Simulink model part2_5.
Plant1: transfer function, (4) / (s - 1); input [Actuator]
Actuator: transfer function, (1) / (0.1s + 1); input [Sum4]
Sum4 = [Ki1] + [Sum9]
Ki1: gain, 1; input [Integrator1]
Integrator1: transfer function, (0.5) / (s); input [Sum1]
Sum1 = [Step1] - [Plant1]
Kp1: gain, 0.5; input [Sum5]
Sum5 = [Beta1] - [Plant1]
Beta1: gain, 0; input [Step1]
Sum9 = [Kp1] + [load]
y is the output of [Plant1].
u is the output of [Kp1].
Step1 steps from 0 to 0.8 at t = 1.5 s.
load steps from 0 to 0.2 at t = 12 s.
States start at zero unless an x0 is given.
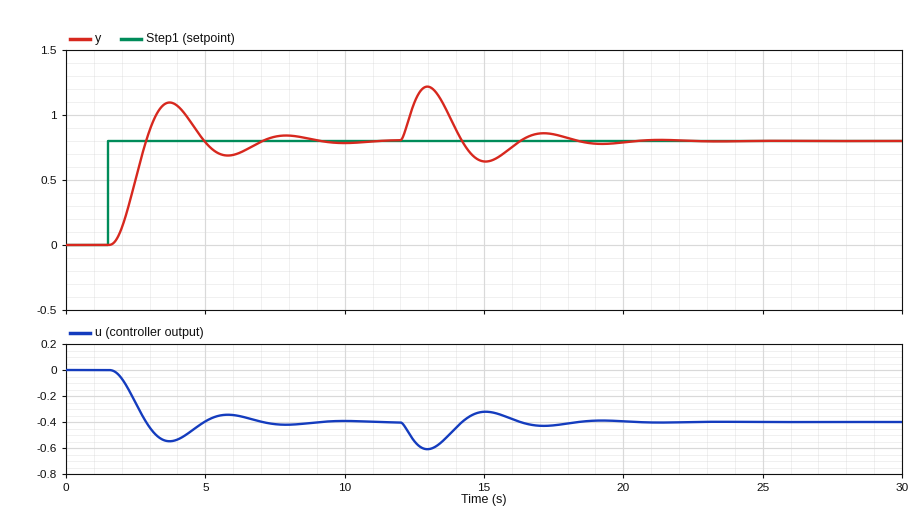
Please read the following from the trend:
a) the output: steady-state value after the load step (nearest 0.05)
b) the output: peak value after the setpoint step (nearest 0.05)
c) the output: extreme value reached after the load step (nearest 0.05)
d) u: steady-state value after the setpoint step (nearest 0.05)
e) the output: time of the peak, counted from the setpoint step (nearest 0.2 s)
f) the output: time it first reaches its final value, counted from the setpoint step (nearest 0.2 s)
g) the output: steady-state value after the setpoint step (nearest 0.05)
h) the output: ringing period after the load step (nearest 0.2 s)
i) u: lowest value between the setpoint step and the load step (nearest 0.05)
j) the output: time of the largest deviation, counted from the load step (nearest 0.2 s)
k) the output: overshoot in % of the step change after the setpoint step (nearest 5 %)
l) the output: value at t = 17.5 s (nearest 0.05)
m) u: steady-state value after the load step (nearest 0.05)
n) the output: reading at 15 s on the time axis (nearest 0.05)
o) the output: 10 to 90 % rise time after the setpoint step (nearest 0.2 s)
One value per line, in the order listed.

0.80
1.10
1.20
-0.40
2.2 s
1.4 s
0.80
4.2 s
-0.55
1.0 s
35 %
0.85
-0.40
0.65
0.8 s
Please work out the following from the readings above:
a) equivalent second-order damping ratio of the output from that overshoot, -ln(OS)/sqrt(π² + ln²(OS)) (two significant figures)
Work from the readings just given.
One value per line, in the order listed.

0.32
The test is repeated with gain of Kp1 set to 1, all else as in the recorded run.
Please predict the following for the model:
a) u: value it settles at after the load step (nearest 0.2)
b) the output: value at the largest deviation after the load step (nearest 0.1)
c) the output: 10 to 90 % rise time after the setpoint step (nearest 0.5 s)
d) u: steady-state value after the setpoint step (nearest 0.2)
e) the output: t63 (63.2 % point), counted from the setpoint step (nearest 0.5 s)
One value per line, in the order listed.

-0.8
1.0
2.5 s
-0.8
1.5 s
